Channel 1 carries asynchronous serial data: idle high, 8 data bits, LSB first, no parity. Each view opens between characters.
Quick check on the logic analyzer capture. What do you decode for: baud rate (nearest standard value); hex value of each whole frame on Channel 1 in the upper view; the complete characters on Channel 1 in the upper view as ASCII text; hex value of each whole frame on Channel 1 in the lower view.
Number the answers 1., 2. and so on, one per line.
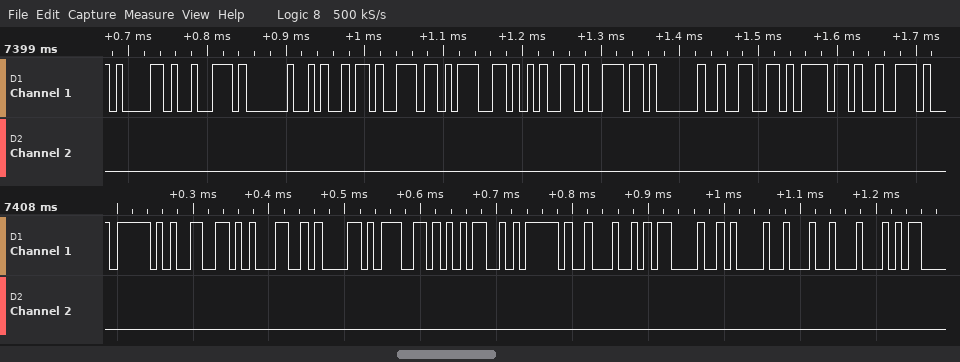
1. 115200 baud
2. 61, 72, 20, 69, 6E, 67, 65, 6E, 20, 66, 6F, 72
3. "ar ingen for"
4. 5F, 66, 31, 61, 67, 35, 7D, 22, 0D, 0A, 22, 44
